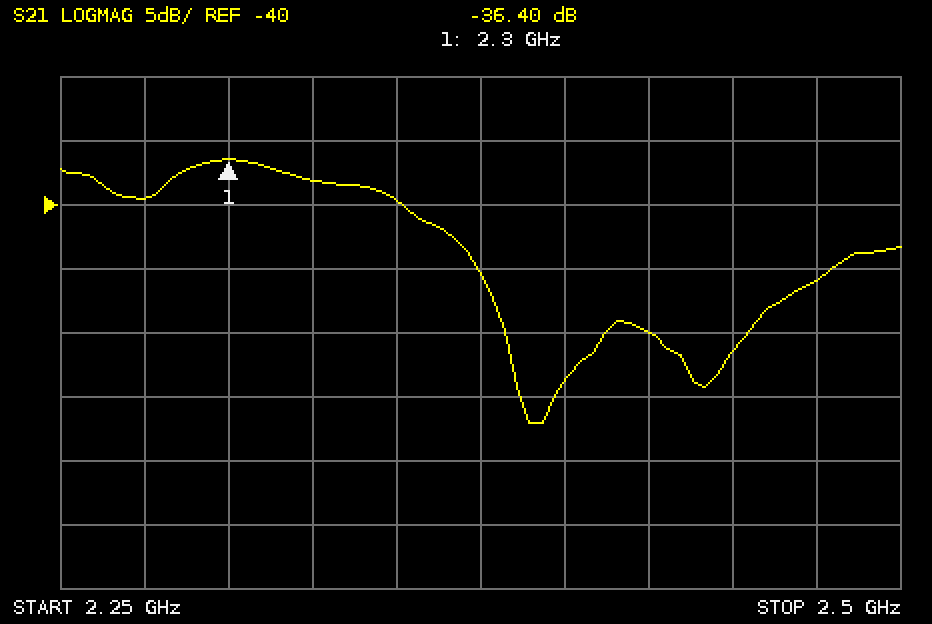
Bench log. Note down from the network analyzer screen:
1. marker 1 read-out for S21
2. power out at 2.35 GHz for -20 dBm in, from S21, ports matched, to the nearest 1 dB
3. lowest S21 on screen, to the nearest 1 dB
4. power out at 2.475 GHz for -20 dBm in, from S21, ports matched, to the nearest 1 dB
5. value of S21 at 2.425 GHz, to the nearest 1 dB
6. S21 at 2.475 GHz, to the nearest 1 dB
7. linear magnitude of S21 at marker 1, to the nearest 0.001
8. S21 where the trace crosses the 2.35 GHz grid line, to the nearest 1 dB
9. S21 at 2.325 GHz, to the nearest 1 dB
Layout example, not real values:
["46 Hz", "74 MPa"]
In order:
["-36.40 dB", "-60 dBm", "-57 dB", "-66 dBm", "-50 dB", "-46 dB", "0.015", "-40 dB", "-38 dB"]
